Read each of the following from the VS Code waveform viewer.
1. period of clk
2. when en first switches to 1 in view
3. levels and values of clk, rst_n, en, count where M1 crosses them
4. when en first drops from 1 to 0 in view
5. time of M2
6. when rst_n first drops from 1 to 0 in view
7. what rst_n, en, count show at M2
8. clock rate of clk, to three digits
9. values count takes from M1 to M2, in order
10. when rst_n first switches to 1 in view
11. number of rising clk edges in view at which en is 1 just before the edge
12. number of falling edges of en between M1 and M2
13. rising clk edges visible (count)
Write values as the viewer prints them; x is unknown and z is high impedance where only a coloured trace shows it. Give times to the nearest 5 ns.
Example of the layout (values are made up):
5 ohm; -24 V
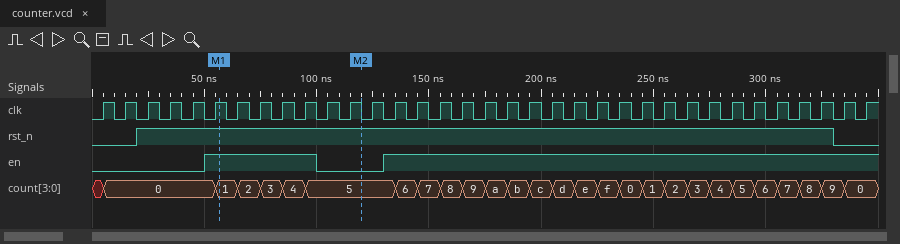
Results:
10 ns; 50 ns; clk=1, rst_n=1, en=1, count=1; 100 ns; 120 ns; 330 ns; rst_n=1, en=0, count=5; 100 MHz; 1, 2, 3, 4, 5; 20 ns; 27; 1; 35
